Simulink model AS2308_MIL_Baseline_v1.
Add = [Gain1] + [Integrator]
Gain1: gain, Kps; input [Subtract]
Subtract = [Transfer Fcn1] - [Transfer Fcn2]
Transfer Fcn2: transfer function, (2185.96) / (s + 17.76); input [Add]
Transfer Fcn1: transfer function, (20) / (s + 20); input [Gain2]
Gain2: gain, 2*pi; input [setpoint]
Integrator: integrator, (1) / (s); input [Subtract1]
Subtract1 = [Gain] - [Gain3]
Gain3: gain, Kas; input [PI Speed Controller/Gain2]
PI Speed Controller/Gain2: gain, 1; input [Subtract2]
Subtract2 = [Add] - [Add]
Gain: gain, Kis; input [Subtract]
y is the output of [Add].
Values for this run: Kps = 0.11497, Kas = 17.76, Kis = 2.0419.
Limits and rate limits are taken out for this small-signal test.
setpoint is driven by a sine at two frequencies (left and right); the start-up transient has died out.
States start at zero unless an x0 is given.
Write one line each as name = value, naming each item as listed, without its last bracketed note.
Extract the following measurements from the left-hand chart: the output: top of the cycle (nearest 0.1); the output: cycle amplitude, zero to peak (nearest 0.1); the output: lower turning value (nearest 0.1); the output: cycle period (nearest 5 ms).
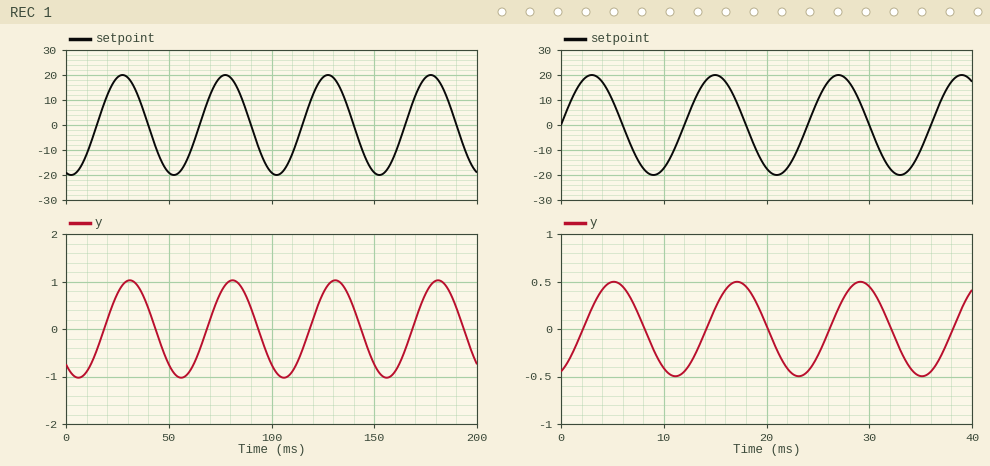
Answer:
the output: top of the cycle = 1.0
the output: cycle amplitude, zero to peak = 1.0
the output: lower turning value = -1.0
the output: cycle period = 50 ms
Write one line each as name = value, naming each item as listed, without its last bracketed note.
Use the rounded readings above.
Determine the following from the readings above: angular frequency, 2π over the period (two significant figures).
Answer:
angular frequency, 2π over the period = 0.13 rad/ms
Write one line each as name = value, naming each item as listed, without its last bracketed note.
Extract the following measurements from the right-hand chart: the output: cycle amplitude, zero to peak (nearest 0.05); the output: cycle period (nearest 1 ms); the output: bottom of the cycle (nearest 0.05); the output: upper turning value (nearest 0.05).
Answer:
the output: cycle amplitude, zero to peak = 0.50
the output: cycle period = 12 ms
the output: bottom of the cycle = -0.50
the output: upper turning value = 0.50
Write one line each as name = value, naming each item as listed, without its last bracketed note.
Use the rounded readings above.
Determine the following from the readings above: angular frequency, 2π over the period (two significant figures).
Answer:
angular frequency, 2π over the period = 0.52 rad/ms
